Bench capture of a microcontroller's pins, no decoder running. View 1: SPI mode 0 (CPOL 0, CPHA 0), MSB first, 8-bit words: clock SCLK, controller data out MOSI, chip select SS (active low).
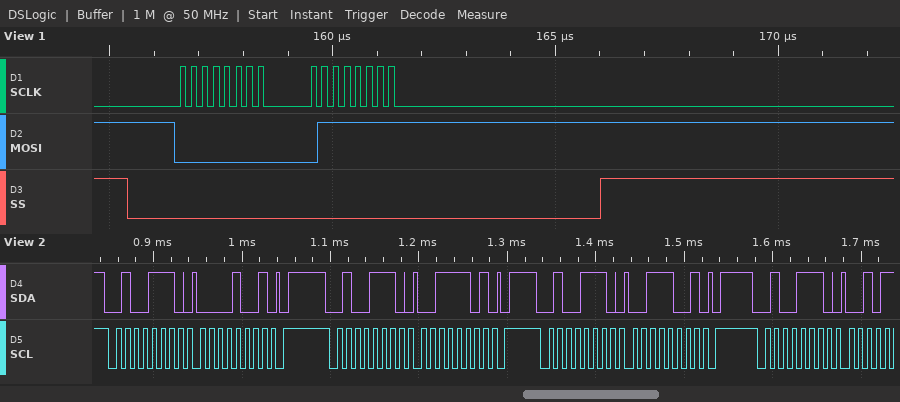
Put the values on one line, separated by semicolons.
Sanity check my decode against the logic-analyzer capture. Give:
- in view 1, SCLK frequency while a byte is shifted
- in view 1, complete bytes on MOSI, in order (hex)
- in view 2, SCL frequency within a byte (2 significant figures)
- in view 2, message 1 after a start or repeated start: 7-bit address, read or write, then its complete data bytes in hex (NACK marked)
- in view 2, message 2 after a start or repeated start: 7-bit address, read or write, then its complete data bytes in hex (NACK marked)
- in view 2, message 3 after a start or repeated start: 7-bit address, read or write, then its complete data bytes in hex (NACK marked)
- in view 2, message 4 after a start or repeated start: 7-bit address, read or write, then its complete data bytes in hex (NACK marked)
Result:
4 MHz; 00 7F; 100 kHz; 0x27 write: 09; 0x27 write: 3D; 0x27 write: 39; 0x27 write
